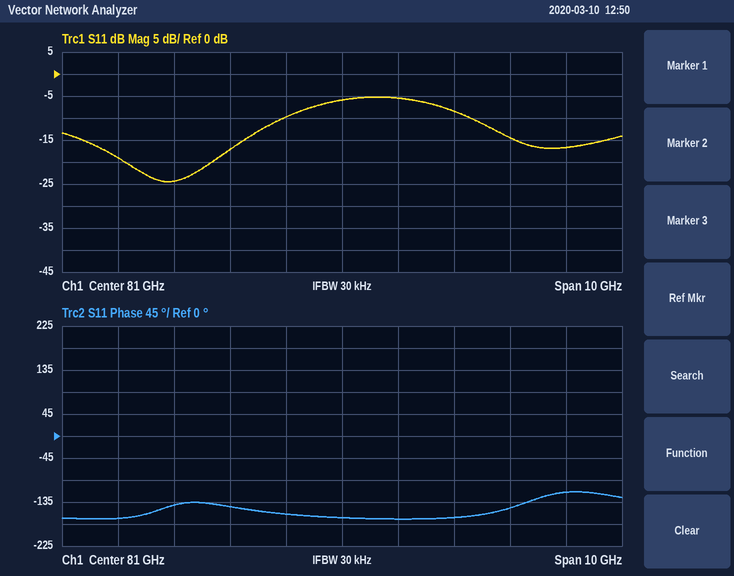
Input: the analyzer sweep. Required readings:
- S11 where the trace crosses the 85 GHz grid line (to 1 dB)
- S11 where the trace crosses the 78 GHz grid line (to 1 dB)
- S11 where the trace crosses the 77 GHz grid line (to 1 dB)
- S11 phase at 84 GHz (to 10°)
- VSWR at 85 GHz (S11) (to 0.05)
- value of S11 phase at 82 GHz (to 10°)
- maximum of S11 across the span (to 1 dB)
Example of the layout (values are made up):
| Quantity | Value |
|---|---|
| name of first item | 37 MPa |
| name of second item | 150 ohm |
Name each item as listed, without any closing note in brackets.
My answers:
| Quantity | Value |
|---|---|
| S11 where the trace crosses the 85 GHz grid line | -17 dB |
| S11 where the trace crosses the 78 GHz grid line | -24 dB |
| S11 where the trace crosses the 77 GHz grid line | -19 dB |
| S11 phase at 84 GHz | -150° |
| VSWR at 85 GHz (S11) | 1.35 |
| value of S11 phase at 82 GHz | -170° |
| maximum of S11 across the span | -5 dB |
